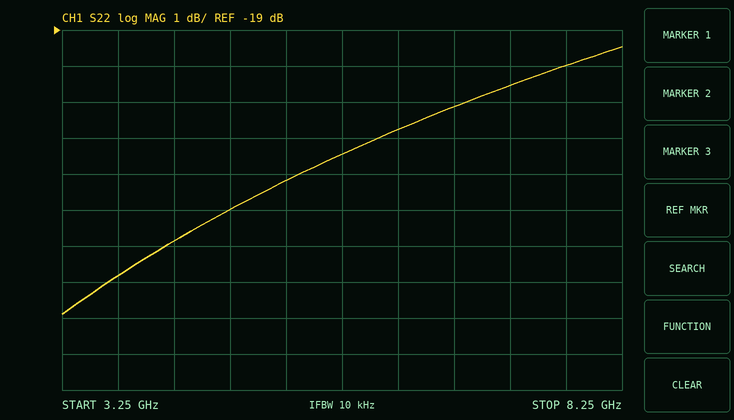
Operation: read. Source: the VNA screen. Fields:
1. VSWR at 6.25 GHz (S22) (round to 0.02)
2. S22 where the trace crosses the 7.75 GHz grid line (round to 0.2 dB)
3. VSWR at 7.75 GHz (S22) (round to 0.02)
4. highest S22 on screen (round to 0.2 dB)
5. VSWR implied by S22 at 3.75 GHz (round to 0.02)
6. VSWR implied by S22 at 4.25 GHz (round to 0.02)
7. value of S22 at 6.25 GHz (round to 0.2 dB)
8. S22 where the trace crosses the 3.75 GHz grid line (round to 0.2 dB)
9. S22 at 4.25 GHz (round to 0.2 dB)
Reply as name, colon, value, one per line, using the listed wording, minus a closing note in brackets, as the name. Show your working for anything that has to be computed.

VSWR at 6.25 GHz (S22): |Γ| = 10^(-21.8/20) = 0.0813; VSWR = (1 + 0.0813)/(1 − 0.0813) ≈ 1.18
S22 where the trace crosses the 7.75 GHz grid line: -20.0 dB
VSWR at 7.75 GHz (S22): |Γ| = 10^(-20/20) = 0.1000; VSWR = (1 + 0.1000)/(1 − 0.1000) ≈ 1.22
highest S22 on screen: -19.4 dB
VSWR implied by S22 at 3.75 GHz: |Γ| = 10^(-25.8/20) = 0.0513; VSWR = (1 + 0.0513)/(1 − 0.0513) ≈ 1.11, so 1.10 to the nearest 0.02
VSWR implied by S22 at 4.25 GHz: |Γ| = 10^(-24.8/20) = 0.0575; VSWR = (1 + 0.0575)/(1 − 0.0575) ≈ 1.12
value of S22 at 6.25 GHz: -21.8 dB
S22 where the trace crosses the 3.75 GHz grid line: -25.8 dB
S22 at 4.25 GHz: -24.8 dB
